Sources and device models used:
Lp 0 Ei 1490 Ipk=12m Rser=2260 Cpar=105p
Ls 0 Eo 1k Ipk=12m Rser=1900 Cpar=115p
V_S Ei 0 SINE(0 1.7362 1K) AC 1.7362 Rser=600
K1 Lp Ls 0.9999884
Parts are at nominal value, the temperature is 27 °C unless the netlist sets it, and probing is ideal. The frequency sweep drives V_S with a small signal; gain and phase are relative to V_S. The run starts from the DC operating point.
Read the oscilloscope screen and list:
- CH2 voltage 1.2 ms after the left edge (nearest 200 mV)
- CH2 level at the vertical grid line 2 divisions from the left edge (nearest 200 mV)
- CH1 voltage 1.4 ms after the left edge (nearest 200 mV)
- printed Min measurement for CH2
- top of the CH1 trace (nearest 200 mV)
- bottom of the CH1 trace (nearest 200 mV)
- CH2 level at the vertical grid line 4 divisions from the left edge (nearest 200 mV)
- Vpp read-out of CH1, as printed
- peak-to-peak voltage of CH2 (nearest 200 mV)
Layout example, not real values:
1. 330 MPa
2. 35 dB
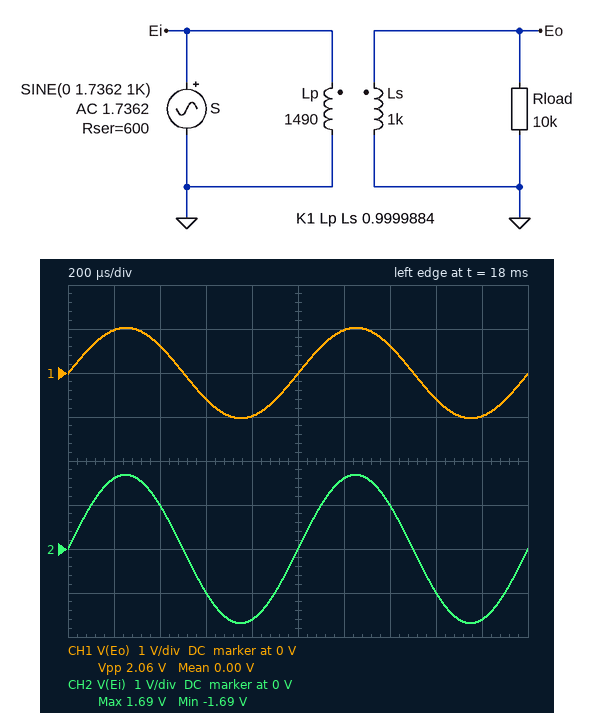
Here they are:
1. 1.6 V
2. 1.0 V
3. 600 mV
4. -1.69 V
5. 1.0 V
6. -1.0 V
7. -1.6 V
8. 2.06 V
9. 3.4 V
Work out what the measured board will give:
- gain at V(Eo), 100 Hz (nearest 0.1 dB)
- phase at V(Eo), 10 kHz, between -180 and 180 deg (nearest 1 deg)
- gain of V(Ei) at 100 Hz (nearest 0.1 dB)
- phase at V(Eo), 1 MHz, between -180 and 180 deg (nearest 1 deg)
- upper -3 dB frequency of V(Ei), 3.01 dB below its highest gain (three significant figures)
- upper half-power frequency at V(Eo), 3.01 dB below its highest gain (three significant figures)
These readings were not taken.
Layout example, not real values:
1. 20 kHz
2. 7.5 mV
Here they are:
1. -4.5 dB
2. -7 deg
3. -0.3 dB
4. 168 deg
5. 2.56 MHz
6. 113 kHz
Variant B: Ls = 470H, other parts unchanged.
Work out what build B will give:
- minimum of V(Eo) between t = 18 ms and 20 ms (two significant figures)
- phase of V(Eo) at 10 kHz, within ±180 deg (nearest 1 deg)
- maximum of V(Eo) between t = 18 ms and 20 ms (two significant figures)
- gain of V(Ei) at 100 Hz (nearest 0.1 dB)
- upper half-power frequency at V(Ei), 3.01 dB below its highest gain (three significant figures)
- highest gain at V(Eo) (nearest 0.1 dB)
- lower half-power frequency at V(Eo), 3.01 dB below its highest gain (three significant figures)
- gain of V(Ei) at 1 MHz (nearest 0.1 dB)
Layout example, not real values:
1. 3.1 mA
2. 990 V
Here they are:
1. -760 mV
2. -4 deg
3. 760 mV
4. -0.1 dB
5. 2.57 MHz
6. -6.5 dB
7. 336 mHz
8. -0.6 dB
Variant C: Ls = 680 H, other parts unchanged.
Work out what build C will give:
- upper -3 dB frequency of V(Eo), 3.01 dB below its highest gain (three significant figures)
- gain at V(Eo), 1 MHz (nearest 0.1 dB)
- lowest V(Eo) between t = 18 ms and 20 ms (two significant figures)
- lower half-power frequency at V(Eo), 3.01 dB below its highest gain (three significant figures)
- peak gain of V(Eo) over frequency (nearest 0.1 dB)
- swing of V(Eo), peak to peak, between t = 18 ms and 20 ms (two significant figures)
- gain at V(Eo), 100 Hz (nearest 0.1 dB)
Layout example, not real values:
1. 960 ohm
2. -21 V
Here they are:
1. 148 kHz
2. -41.1 dB
3. -890 mV
4. 288 mHz
5. -5.6 dB
6. 1.8 V
7. -5.8 dB
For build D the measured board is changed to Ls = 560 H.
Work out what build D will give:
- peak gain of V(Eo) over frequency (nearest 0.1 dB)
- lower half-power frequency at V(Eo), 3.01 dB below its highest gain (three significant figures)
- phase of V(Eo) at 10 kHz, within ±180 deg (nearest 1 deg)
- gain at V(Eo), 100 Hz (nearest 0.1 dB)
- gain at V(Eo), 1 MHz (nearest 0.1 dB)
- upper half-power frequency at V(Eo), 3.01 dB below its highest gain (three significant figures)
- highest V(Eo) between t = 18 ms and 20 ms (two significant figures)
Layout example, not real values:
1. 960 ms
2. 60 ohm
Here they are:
1. -6.1 dB
2. 310 mHz
3. -5 deg
4. -6.5 dB
5. -40.2 dB
6. 166 kHz
7. 820 mV
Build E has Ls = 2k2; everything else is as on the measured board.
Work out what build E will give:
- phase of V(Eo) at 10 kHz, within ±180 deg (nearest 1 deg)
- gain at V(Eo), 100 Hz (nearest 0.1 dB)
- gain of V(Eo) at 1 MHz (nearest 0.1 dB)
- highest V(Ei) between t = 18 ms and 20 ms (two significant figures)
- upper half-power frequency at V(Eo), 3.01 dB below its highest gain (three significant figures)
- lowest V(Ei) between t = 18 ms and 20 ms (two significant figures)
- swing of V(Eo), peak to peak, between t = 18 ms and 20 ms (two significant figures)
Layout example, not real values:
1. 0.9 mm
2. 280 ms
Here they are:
1. -13 deg
2. -2.5 dB
3. -46.3 dB
4. 1.6 V
5. 58.3 kHz
6. -1.6 V
7. 2.6 V
